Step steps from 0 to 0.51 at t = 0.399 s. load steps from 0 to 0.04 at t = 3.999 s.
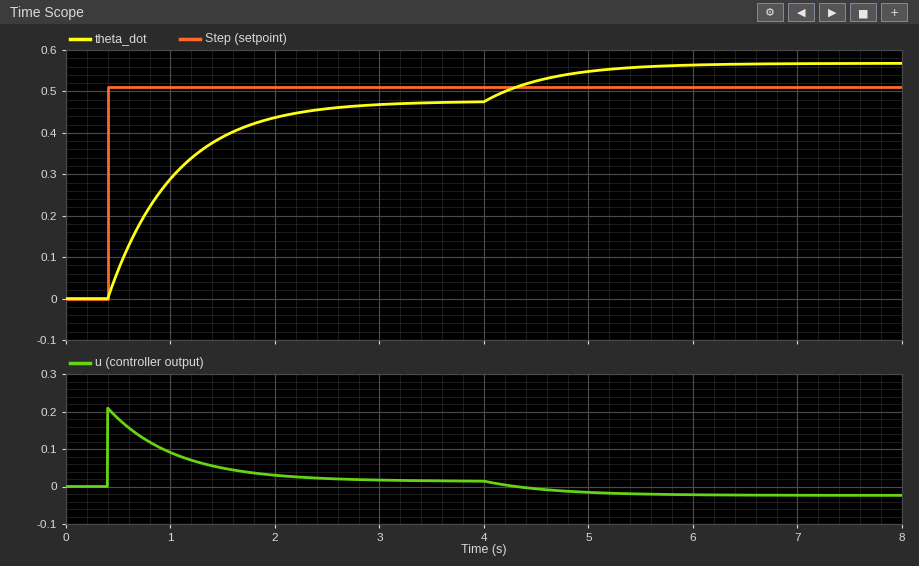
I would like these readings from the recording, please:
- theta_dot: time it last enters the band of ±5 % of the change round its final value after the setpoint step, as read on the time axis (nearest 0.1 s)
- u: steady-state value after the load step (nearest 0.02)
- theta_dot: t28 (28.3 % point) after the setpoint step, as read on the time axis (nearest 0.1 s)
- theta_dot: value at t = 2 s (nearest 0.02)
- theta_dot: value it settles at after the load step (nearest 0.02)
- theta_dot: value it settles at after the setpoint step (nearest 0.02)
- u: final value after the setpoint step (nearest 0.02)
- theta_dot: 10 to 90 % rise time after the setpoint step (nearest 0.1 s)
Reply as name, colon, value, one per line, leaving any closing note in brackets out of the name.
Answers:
theta_dot: time it last enters the band of ±5 % of the change round its final value after the setpoint step, as read on the time axis: 2.3 s
u: steady-state value after the load step: -0.02
theta_dot: t28 (28.3 % point) after the setpoint step, as read on the time axis: 0.6 s
theta_dot: value at t = 2 s: 0.44
theta_dot: value it settles at after the load step: 0.56
theta_dot: value it settles at after the setpoint step: 0.48
u: final value after the setpoint step: 0.02
theta_dot: 10 to 90 % rise time after the setpoint step: 1.4 s
